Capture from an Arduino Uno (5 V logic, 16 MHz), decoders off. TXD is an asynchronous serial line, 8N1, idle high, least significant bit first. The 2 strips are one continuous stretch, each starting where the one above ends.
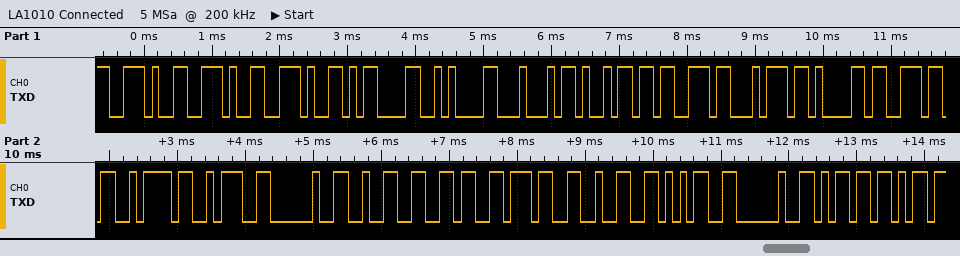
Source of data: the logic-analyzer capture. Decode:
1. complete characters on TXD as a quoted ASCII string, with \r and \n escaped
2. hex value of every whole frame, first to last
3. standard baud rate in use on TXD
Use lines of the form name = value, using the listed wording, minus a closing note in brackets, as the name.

complete characters on TXD as a quoted ASCII string, with \r and \n escaped = "...\r\nDistanz: 26725 m"
hex value of every whole frame, first to last = 2E 2E 2E 0D 0A 44 69 73 74 61 6E 7A 3A 20 32 36 37 32 35 20 6D
standard baud rate in use on TXD = 9600 baud
